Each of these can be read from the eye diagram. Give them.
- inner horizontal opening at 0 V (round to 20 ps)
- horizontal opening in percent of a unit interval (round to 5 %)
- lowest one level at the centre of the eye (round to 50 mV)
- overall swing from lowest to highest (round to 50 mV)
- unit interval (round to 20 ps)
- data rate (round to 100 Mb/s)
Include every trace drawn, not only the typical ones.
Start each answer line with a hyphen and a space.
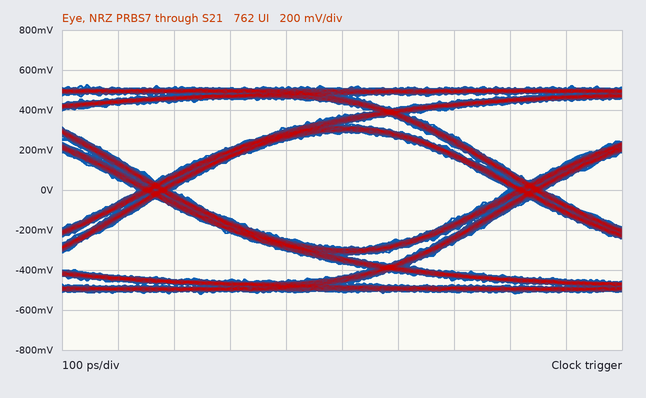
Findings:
- 600 ps
- 90 %
- 300 mV
- 1.05 V
- 660 ps
- 1.5 Gb/s
